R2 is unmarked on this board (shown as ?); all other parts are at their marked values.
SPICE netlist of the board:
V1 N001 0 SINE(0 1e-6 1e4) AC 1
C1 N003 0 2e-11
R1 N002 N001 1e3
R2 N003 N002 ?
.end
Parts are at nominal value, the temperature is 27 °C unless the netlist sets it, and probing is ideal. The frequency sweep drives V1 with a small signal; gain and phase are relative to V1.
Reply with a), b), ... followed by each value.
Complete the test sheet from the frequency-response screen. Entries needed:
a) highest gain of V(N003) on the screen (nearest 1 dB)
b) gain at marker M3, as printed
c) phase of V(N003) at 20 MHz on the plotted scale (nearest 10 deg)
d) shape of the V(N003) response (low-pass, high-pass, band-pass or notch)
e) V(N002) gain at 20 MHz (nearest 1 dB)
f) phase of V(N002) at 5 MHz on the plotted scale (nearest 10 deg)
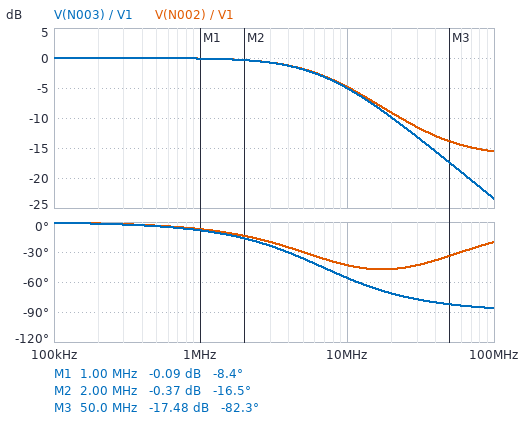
a) 0 dB
b) -17.48 dB
c) -70 deg
d) low-pass
e) -9 dB
f) -30 deg
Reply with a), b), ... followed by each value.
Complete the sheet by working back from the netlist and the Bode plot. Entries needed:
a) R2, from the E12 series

a) 180 Ω
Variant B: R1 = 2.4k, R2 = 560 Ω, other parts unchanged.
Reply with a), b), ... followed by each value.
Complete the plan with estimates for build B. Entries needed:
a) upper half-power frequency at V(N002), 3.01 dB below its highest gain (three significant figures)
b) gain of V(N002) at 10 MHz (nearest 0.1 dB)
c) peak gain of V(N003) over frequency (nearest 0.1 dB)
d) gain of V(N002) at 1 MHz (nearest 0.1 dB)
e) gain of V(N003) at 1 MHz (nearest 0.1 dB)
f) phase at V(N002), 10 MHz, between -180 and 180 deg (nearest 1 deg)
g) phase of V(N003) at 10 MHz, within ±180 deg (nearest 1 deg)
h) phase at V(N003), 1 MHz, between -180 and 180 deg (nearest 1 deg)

a) 2.79 MHz
b) -10.0 dB
c) 0 dB
d) -0.5 dB
e) -0.6 dB
f) -40 deg
g) -75 deg
h) -20 deg
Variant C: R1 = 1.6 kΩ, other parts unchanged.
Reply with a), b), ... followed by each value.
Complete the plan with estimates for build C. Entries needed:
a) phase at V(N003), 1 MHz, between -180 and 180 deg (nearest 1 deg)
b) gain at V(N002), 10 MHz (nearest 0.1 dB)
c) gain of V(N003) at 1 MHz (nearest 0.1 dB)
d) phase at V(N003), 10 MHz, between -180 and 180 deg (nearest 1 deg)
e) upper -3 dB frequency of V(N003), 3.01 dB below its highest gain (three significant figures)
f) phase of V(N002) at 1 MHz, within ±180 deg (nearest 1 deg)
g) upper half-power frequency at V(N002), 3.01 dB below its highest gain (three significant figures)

a) -13 deg
b) -7.6 dB
c) -0.2 dB
d) -66 deg
e) 4.47 MHz
f) -11 deg
g) 4.52 MHz
